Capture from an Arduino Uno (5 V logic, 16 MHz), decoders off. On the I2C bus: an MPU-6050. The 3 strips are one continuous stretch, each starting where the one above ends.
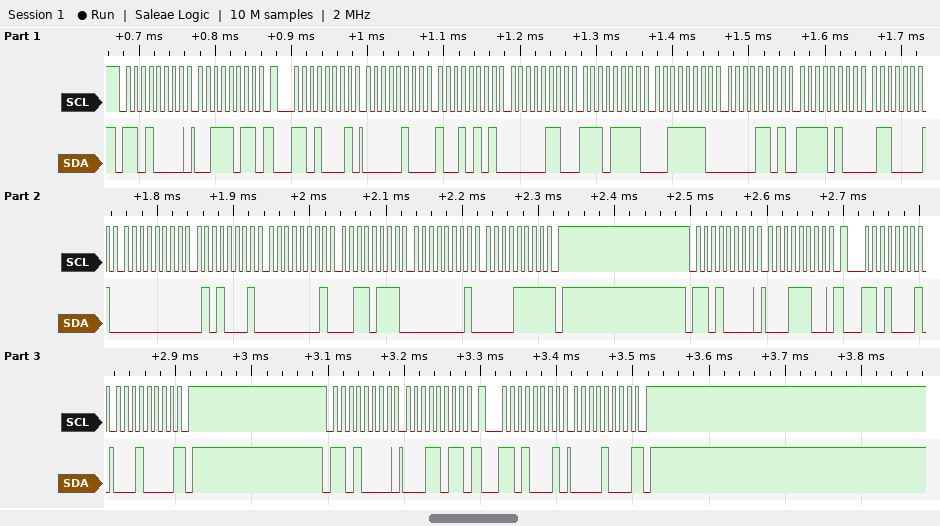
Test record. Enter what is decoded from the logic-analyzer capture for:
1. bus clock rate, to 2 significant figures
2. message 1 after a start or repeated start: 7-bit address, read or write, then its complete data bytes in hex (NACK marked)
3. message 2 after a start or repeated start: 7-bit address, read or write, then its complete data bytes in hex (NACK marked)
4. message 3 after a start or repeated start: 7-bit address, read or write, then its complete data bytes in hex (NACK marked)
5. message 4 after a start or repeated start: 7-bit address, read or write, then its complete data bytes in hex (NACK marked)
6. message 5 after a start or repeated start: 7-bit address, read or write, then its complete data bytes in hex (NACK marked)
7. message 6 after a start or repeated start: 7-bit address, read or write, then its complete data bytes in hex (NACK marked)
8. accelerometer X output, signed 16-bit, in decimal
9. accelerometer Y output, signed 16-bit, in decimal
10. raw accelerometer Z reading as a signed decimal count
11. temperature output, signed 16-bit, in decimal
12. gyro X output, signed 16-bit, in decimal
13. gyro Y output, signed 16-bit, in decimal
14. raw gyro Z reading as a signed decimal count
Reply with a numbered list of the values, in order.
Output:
1. 100 kHz
2. 0x68 write: 3B
3. 0x68 read: 04 95 06 EF 3E 0D F4 61 00 51 01 37 01 0F NACK
4. 0x68 write: 1C
5. 0x68 read: 10 NACK
6. 0x68 write: 1B
7. 0x68 read: 08 NACK
8. 1173
9. 1775
10. 15885
11. -2975
12. 81
13. 311
14. 271
